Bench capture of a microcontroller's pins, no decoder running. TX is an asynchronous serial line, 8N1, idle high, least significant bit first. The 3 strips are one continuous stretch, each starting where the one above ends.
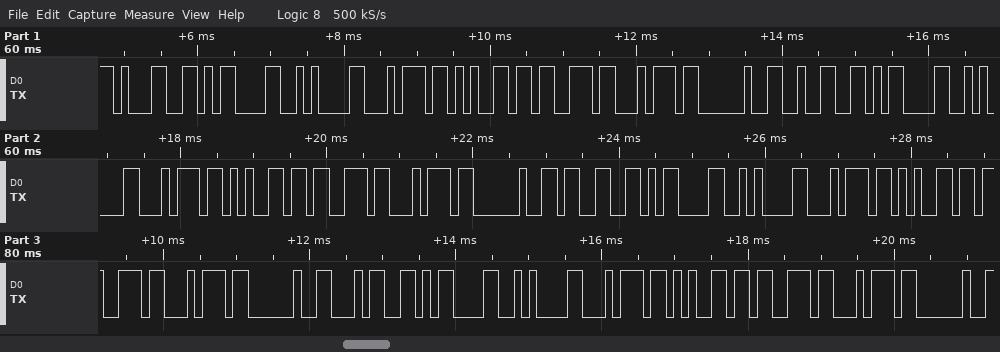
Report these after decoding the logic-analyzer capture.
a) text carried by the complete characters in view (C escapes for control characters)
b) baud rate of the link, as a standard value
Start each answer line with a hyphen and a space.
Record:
- "1\r\ntest 2\r\ntest 3\r\ntest 4\r\ntest "
- 9600 baud
